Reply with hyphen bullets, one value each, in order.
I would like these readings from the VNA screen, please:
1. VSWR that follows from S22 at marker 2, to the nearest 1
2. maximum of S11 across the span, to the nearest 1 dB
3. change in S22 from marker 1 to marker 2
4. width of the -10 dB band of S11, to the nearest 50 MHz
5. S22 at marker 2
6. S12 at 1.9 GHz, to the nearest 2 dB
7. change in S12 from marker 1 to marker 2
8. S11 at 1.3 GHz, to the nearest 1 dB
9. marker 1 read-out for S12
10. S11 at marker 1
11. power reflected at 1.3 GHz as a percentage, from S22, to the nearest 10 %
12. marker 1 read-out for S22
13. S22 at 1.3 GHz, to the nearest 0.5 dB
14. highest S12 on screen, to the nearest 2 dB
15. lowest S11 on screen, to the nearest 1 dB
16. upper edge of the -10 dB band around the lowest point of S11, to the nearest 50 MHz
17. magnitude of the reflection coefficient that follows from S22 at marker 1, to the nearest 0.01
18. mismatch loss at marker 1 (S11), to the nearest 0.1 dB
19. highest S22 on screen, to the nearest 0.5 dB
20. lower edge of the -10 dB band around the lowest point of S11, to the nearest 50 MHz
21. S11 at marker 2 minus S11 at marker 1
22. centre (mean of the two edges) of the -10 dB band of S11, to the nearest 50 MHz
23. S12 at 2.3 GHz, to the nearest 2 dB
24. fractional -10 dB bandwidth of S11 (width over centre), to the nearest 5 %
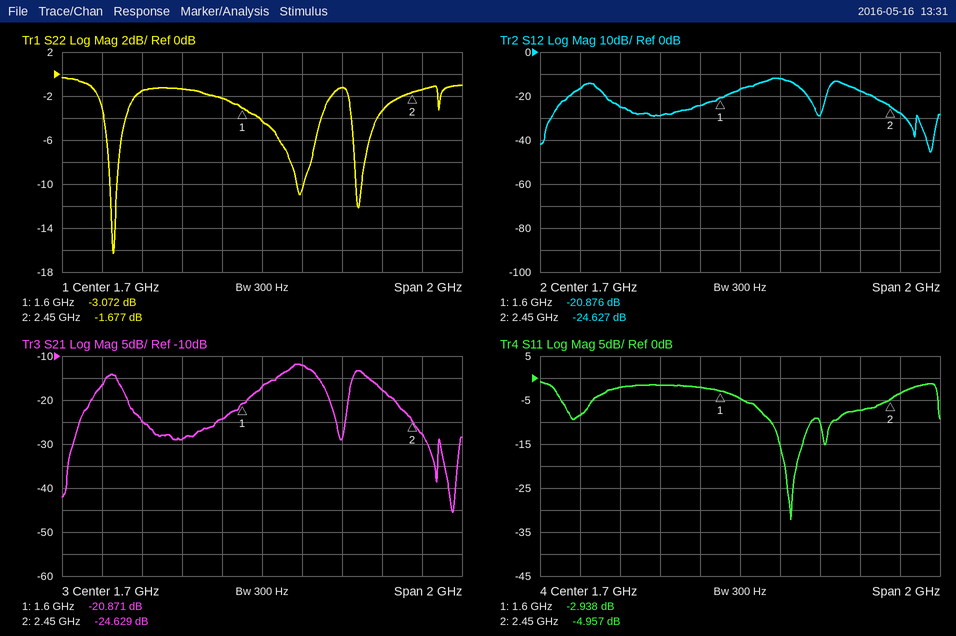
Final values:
- 10
- -1 dB
- 1.395 dB
- 200 MHz
- -1.677 dB
- -12 dB
- -3.751 dB
- -2 dB
- -20.876 dB
- -2.938 dB
- 70 %
- -3.072 dB
- -1.5 dB
- -12 dB
- -32 dB
- 2.05 GHz
- 0.70
- 3.1 dB
- -0.5 dB
- 1.85 GHz
- -2.019 dB
- 1.95 GHz
- -18 dB
- 10 %
